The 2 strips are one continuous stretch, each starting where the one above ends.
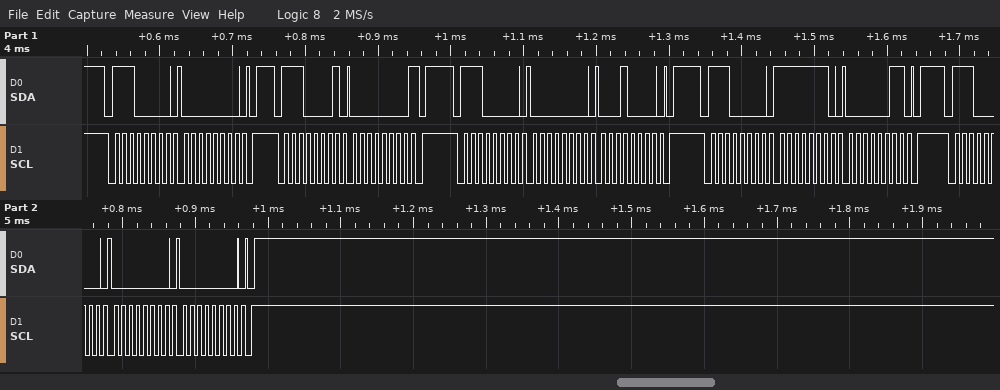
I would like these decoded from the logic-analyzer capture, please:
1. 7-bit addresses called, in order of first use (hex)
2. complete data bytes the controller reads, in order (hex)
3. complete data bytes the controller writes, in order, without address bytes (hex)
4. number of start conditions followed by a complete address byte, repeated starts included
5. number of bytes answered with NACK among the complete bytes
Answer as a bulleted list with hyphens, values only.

- 0x70
- 00
- 00 00 10 FE 03 00 00
- 5
- 1
